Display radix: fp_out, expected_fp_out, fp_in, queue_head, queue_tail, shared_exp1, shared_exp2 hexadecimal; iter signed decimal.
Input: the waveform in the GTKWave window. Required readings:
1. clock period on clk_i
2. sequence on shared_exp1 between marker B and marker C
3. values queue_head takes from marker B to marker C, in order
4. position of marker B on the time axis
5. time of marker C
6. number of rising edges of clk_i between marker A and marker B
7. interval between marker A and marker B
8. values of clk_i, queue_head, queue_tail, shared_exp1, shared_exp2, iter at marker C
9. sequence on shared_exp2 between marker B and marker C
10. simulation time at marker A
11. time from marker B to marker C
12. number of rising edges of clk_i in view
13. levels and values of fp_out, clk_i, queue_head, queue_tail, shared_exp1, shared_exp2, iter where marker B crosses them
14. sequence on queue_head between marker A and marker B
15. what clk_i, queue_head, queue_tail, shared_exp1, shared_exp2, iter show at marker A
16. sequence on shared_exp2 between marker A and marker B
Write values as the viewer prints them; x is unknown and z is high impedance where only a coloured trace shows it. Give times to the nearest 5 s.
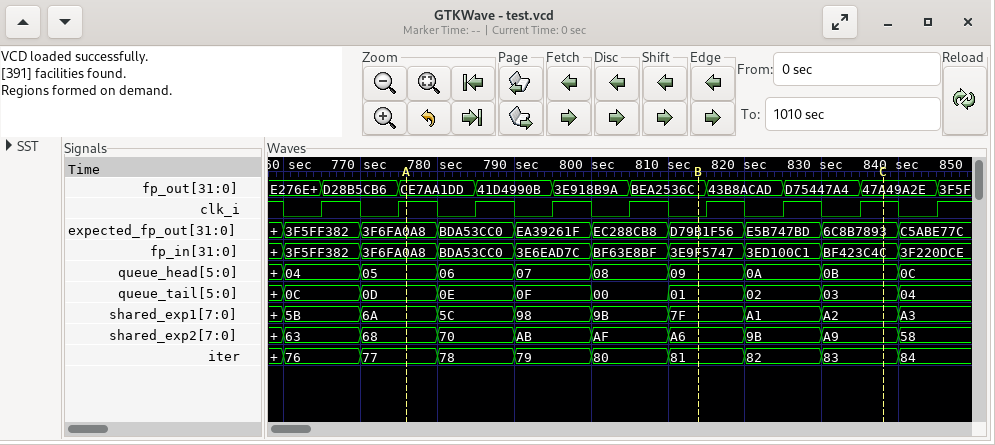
10 s
7F, A1, A2
09, 0A, 0B
815 s
840 s
3
40 s
clk_i=1, queue_head=0B, queue_tail=03, shared_exp1=A2, shared_exp2=A9, iter=83
A6, 9B, A9
775 s
25 s
9
fp_out=BEA2536C, clk_i=0, queue_head=09, queue_tail=01, shared_exp1=7F, shared_exp2=A6, iter=81
05, 06, 07, 08, 09
clk_i=1, queue_head=05, queue_tail=0D, shared_exp1=6A, shared_exp2=68, iter=77
68, 70, AB, AF, A6
